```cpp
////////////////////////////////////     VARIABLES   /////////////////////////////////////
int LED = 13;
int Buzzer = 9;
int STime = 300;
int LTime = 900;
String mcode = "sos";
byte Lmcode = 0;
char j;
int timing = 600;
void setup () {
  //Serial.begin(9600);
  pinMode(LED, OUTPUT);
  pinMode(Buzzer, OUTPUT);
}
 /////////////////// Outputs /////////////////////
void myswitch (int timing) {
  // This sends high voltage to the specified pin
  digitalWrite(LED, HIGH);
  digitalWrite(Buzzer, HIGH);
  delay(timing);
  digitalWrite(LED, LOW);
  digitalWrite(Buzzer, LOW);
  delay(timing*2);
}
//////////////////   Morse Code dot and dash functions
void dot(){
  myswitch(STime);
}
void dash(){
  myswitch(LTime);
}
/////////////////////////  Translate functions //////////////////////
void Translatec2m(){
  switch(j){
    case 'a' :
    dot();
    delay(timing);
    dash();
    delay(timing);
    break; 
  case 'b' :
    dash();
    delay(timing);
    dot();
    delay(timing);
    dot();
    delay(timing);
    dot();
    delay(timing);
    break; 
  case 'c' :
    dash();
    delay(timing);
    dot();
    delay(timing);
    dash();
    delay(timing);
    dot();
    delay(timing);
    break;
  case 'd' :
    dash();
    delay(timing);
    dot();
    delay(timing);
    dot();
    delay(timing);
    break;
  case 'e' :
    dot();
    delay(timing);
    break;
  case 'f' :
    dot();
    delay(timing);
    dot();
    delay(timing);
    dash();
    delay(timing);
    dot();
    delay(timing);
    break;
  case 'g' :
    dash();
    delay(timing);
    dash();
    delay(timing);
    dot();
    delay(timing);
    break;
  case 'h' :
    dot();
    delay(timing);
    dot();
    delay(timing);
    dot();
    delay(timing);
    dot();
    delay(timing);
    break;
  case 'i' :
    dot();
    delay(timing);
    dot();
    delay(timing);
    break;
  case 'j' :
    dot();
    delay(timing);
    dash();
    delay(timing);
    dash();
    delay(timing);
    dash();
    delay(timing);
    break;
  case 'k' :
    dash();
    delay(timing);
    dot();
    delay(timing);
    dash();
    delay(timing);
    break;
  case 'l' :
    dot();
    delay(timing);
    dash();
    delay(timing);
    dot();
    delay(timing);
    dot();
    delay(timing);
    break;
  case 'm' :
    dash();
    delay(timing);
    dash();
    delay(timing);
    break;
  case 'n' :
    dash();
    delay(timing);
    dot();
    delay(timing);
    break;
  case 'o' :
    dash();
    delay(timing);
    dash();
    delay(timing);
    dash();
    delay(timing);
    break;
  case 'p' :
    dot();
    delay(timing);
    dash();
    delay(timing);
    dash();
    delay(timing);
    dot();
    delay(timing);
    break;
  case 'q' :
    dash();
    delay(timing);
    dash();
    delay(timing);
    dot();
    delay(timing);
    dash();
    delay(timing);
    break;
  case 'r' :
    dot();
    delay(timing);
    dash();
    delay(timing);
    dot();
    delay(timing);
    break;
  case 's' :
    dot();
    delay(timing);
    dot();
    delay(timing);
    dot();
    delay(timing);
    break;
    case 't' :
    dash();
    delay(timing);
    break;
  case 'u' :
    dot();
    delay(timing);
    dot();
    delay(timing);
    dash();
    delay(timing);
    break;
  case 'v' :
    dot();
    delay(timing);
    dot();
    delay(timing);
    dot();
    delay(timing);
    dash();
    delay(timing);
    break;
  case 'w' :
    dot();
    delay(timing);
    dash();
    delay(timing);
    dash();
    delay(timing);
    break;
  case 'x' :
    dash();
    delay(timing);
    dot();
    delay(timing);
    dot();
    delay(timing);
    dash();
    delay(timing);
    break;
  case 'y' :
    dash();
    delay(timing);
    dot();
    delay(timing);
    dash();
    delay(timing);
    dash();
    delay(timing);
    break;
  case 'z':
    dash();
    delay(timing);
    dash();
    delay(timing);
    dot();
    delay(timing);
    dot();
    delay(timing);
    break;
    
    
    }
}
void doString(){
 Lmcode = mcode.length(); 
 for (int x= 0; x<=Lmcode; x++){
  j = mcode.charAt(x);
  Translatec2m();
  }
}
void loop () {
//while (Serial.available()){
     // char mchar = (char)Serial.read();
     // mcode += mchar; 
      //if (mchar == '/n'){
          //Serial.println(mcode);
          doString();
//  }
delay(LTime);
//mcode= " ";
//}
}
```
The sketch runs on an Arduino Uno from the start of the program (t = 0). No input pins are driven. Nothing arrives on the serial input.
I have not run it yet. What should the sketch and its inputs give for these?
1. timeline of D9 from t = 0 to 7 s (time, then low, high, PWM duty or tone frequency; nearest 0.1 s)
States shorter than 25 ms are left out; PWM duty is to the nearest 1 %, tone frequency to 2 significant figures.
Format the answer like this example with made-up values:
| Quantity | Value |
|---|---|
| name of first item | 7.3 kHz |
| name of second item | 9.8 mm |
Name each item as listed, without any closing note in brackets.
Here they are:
| Quantity | Value |
|---|---|
| timeline of D9 from t = 0 to 7 s | 0 s high; 0.3 s low; 1.5 s high; 1.8 s low; 3 s high; 3.3 s low; 4.5 s high; 5.4 s low |
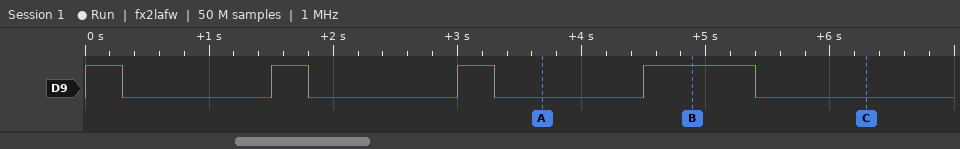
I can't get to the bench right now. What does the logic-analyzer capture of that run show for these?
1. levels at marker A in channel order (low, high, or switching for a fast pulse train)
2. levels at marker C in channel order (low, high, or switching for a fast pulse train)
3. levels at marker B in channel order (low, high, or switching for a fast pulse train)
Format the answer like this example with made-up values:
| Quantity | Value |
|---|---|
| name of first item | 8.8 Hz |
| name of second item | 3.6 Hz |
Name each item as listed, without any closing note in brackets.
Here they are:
| Quantity | Value |
|---|---|
| levels at marker A in channel order | D9 low |
| levels at marker C in channel order | D9 low |
| levels at marker B in channel order | D9 high |
